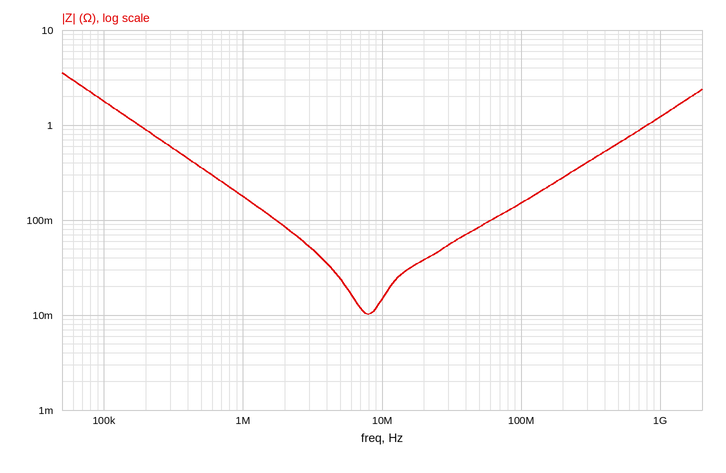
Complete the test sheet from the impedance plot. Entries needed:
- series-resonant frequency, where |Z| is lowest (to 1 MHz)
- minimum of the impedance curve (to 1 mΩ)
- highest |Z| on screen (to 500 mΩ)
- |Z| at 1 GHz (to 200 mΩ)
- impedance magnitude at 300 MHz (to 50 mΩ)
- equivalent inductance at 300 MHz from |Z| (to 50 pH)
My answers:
8 MHz
10 mΩ
3.5 Ω
1.2 Ω
400 mΩ
200 pH
